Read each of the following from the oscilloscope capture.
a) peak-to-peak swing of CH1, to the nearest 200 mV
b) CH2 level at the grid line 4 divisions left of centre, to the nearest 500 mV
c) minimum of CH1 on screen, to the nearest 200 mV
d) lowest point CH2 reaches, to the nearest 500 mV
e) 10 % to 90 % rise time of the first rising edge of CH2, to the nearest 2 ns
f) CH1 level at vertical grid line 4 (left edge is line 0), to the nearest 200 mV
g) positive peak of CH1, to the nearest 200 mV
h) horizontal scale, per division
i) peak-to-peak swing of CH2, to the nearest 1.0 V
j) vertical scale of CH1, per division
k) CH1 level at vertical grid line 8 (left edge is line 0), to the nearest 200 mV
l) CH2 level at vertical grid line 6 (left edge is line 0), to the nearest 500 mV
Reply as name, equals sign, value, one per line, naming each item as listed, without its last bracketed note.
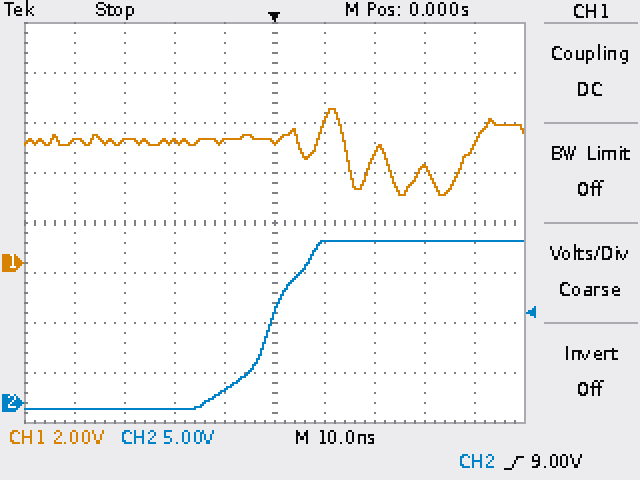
peak-to-peak swing of CH1, to the nearest 200 mV = 3.4 V
CH2 level at the grid line 4 divisions left of centre, to the nearest 500 mV = -500 mV
minimum of CH1 on screen, to the nearest 200 mV = 2.8 V
lowest point CH2 reaches, to the nearest 500 mV = -500 mV
10 % to 90 % rise time of the first rising edge of CH2, to the nearest 2 ns = 18 ns
CH1 level at vertical grid line 4 (left edge is line 0), to the nearest 200 mV = 4.8 V
positive peak of CH1, to the nearest 200 mV = 6.2 V
horizontal scale, per division = 10 ns
peak-to-peak swing of CH2, to the nearest 1.0 V = 17.0 V
vertical scale of CH1, per division = 2 V
CH1 level at vertical grid line 8 (left edge is line 0), to the nearest 200 mV = 3.8 V
CH2 level at vertical grid line 6 (left edge is line 0), to the nearest 500 mV = 16.0 V
